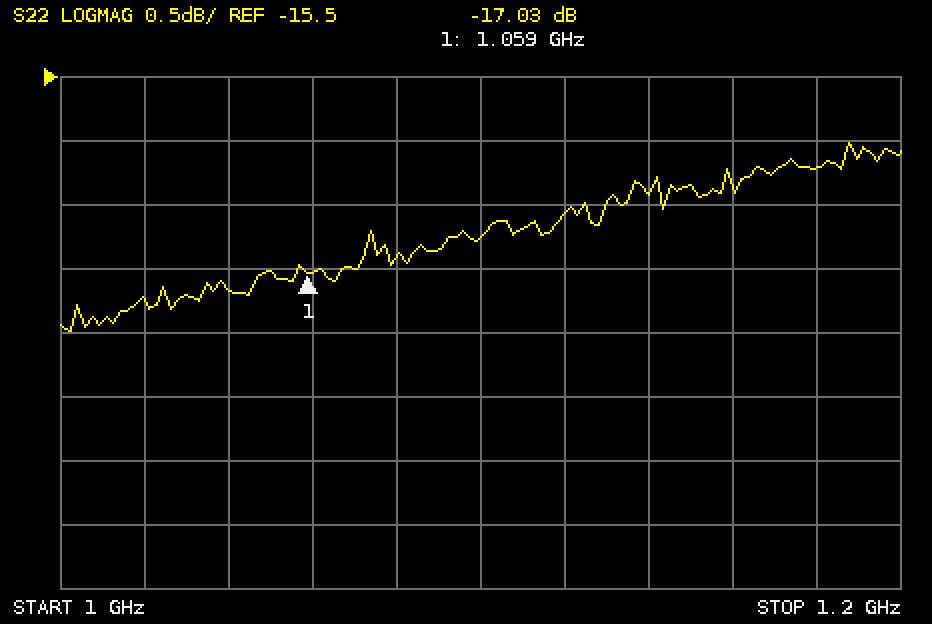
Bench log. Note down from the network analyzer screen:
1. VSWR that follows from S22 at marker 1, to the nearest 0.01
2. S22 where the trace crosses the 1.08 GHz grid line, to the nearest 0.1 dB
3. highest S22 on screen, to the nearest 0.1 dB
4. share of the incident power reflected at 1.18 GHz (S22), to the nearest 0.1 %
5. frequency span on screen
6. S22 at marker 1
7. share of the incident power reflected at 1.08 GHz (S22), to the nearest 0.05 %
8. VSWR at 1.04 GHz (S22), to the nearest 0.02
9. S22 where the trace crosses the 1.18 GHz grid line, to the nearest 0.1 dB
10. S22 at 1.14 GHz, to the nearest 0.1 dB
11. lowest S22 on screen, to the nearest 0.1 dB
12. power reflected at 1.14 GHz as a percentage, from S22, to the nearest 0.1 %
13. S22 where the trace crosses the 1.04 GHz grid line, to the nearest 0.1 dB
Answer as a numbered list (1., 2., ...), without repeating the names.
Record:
1. 1.33
2. -16.9 dB
3. -16.0 dB
4. 2.4 %
5. 200 MHz
6. -17.03 dB
7. 2.05 %
8. 1.32
9. -16.2 dB
10. -16.4 dB
11. -17.5 dB
12. 2.3 %
13. -17.2 dB
